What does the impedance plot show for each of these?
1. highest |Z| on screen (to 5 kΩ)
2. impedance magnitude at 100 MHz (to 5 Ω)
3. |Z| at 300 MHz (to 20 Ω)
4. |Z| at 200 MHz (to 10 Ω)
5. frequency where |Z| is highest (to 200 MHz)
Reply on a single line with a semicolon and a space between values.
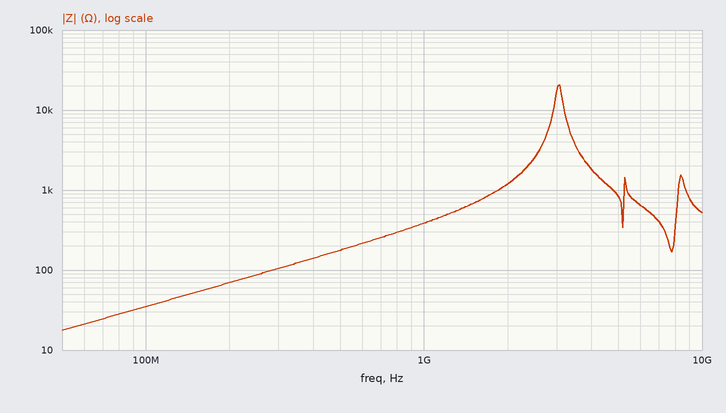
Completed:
20 kΩ; 35 Ω; 100 Ω; 70 Ω; 3.0 GHz
